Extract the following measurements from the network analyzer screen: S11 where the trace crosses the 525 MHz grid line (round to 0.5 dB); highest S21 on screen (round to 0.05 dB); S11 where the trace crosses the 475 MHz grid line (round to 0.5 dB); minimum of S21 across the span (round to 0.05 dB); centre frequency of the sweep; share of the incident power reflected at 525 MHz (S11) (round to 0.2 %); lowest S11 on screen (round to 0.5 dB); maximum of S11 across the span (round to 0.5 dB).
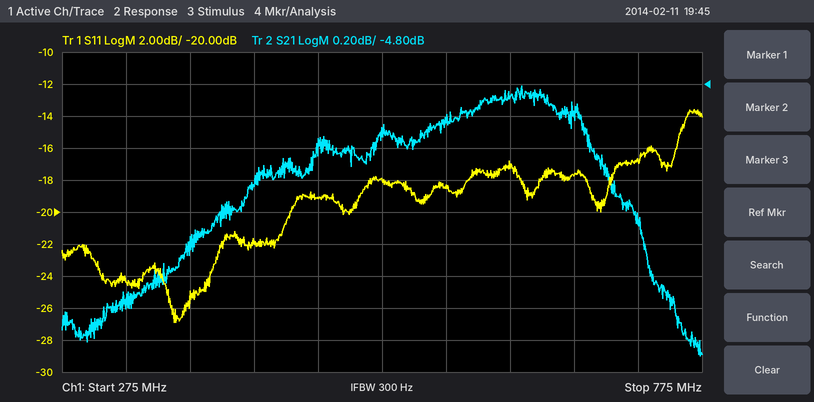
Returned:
-18.0 dB
-4.80 dB
-19.0 dB
-6.50 dB
525 MHz
1.6 %
-27.0 dB
-13.5 dB
